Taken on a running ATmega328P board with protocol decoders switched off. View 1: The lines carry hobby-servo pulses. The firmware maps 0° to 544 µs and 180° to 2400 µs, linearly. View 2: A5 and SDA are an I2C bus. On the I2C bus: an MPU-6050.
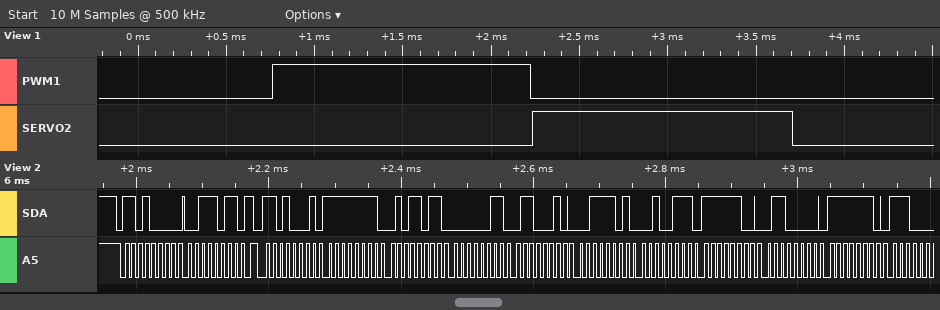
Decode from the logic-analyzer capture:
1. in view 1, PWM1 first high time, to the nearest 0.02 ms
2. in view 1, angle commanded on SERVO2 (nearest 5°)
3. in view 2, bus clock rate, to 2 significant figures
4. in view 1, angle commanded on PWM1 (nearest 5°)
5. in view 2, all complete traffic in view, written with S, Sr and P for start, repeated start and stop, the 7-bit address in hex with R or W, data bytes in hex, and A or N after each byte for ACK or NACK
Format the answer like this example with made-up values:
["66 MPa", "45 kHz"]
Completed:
["1.46 ms", "90°", "100 kHz", "90°", "S 68W A 3B A Sr 68R A FF A 5B A 03 A 62 A 3D A 27 A FC A 60 A FE A"]
